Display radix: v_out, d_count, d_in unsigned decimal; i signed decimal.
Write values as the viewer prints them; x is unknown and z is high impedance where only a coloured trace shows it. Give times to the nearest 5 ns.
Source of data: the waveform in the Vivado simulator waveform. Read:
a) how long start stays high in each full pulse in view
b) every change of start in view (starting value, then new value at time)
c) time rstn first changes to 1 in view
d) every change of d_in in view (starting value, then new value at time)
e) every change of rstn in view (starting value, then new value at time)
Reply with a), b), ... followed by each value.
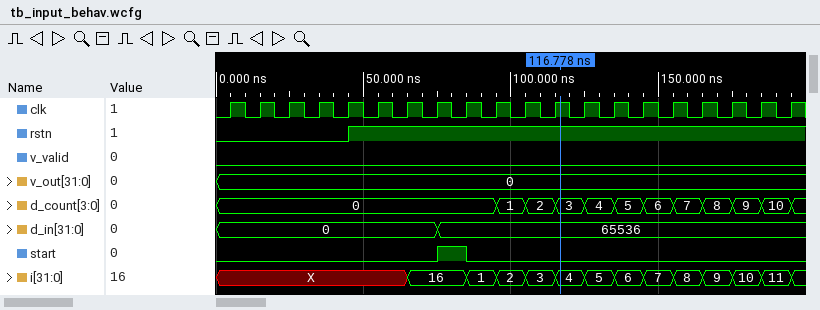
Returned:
a) 10 ns
b) 0, 1 at 75 ns, 0 at 85 ns
c) 45 ns
d) 0, 65536 at 75 ns
e) 0, 1 at 45 ns
